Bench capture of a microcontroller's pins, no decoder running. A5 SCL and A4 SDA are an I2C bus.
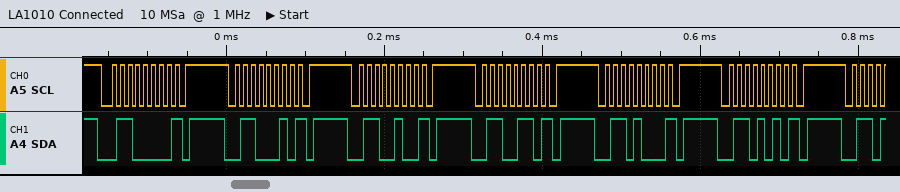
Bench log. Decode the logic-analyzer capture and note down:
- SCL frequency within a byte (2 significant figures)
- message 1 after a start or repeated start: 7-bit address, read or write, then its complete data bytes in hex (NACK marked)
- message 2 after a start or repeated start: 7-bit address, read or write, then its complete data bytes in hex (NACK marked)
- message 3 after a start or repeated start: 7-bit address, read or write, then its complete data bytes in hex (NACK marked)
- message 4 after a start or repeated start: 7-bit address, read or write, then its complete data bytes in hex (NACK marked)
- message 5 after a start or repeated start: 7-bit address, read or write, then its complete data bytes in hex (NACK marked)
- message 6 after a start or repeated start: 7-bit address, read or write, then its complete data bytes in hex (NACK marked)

100 kHz
0x30 write NACK
0x31 write NACK
0x32 write NACK
0x33 write NACK
0x34 write NACK
0x35 write NACK
